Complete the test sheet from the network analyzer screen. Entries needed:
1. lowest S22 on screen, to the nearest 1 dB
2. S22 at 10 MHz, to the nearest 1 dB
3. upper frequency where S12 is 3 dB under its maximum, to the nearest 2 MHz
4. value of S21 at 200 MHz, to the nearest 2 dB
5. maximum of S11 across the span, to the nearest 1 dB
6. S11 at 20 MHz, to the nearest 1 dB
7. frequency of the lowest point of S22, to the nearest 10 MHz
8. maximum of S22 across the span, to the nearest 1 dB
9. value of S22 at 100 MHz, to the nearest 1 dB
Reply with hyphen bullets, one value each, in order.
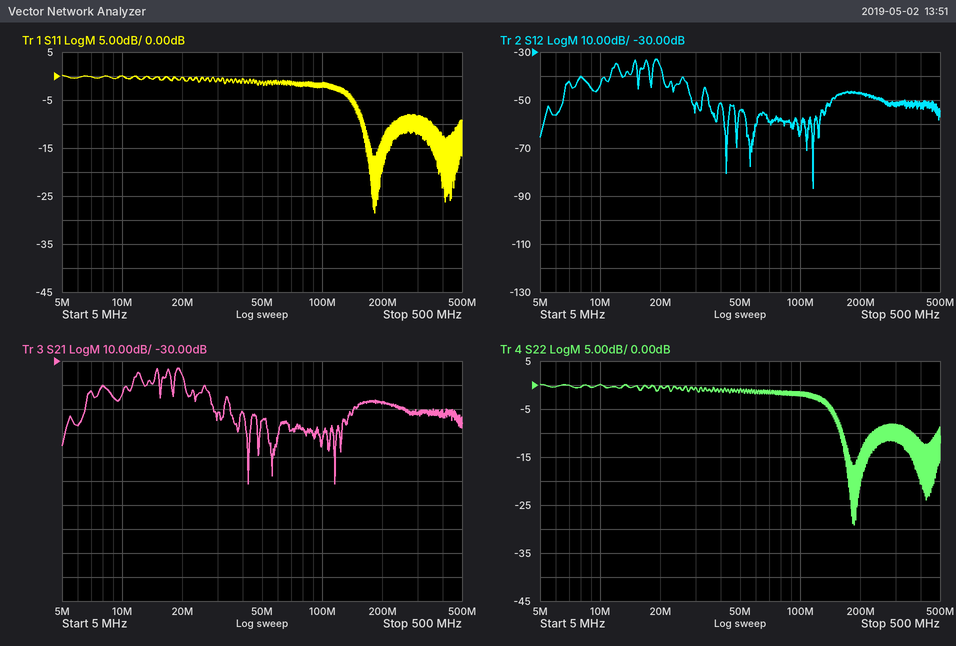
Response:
- -29 dB
- 0 dB
- 20 MHz
- -48 dB
- 0 dB
- 0 dB
- 190 MHz
- 0 dB
- -2 dB
